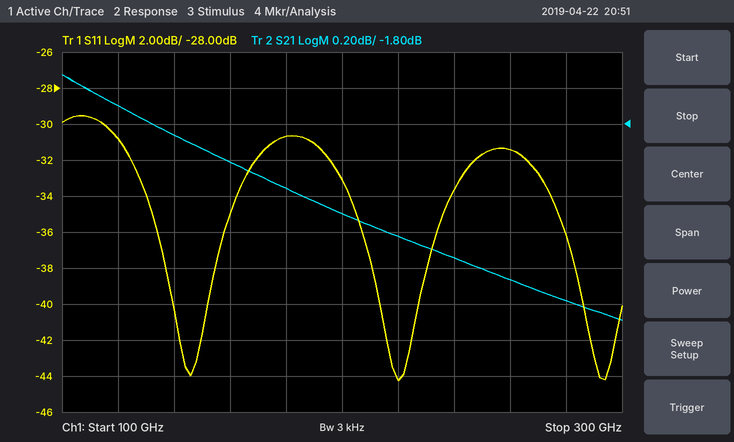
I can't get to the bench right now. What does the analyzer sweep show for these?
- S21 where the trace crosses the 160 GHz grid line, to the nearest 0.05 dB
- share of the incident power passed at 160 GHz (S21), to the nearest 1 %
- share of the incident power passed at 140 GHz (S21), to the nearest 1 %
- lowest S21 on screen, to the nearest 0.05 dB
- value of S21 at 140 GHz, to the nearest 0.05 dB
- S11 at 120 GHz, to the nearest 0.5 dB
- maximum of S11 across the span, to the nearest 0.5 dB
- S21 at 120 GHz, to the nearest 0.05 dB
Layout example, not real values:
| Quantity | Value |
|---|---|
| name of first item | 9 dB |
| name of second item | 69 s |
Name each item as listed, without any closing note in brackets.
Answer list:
| Quantity | Value |
|---|---|
| S21 where the trace crosses the 160 GHz grid line, to the nearest 0.05 dB | -2.00 dB |
| share of the incident power passed at 160 GHz (S21), to the nearest 1 % | 63 % |
| share of the incident power passed at 140 GHz (S21), to the nearest 1 % | 65 % |
| lowest S21 on screen, to the nearest 0.05 dB | -2.90 dB |
| value of S21 at 140 GHz, to the nearest 0.05 dB | -1.85 dB |
| S11 at 120 GHz, to the nearest 0.5 dB | -31.0 dB |
| maximum of S11 across the span, to the nearest 0.5 dB | -29.5 dB |
| S21 at 120 GHz, to the nearest 0.05 dB | -1.70 dB |
